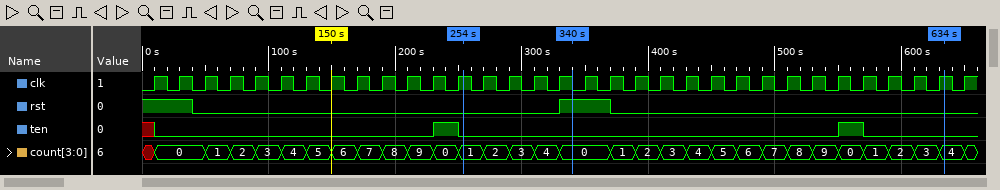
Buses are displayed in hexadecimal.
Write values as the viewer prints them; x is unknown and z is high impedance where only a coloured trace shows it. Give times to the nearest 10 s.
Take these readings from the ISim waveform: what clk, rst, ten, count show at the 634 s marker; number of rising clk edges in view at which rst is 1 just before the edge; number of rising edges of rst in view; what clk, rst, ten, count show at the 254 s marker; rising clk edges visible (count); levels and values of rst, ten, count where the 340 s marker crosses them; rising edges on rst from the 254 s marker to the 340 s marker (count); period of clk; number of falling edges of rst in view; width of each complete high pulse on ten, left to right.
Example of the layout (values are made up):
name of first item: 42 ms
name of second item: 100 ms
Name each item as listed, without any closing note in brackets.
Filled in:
what clk, rst, ten, count show at the 634 s marker: clk=1, rst=0, ten=0, count=4
number of rising clk edges in view at which rst is 1 just before the edge: 4
number of rising edges of rst in view: 1
what clk, rst, ten, count show at the 254 s marker: clk=1, rst=0, ten=0, count=1
rising clk edges visible: 33
levels and values of rst, ten, count where the 340 s marker crosses them: rst=1, ten=0, count=0
rising edges on rst from the 254 s marker to the 340 s marker: 1
period of clk: 20 s
number of falling edges of rst in view: 2
width of each complete high pulse on ten, left to right: 20 s, 20 s
